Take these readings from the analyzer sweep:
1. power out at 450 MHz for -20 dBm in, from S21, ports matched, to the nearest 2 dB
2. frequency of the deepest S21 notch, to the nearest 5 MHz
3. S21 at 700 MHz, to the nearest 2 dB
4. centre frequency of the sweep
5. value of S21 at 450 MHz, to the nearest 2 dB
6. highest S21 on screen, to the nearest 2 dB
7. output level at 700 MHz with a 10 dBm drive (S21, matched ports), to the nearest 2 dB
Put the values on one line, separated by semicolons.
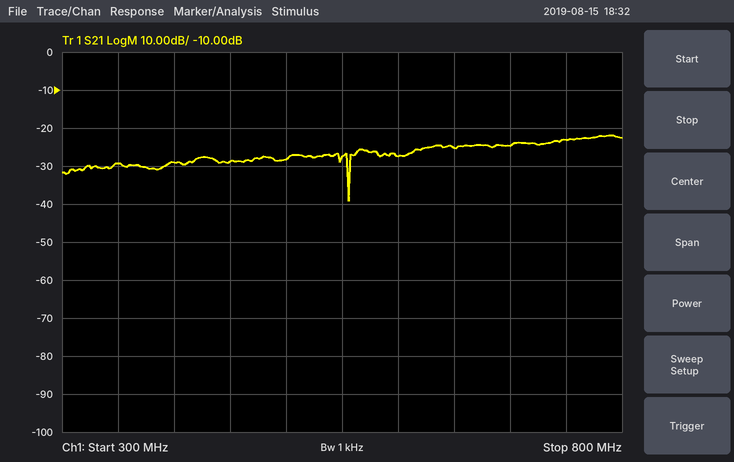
-48 dBm; 555 MHz; -24 dB; 550 MHz; -28 dB; -22 dB; -14 dBm
